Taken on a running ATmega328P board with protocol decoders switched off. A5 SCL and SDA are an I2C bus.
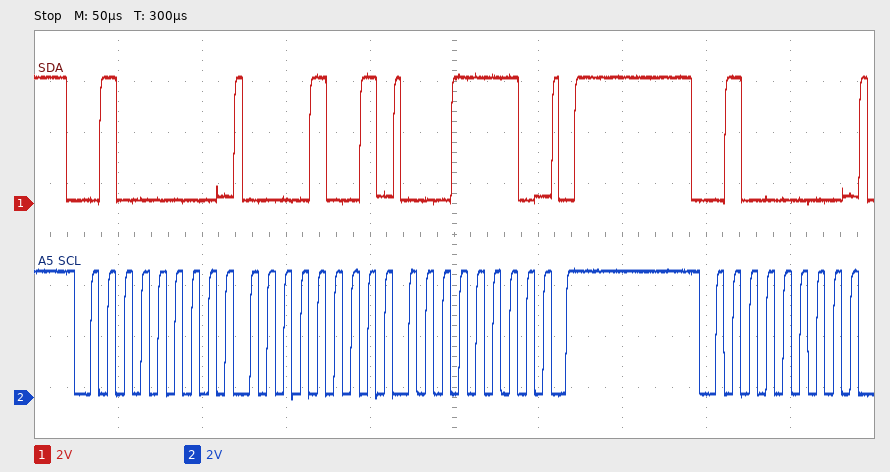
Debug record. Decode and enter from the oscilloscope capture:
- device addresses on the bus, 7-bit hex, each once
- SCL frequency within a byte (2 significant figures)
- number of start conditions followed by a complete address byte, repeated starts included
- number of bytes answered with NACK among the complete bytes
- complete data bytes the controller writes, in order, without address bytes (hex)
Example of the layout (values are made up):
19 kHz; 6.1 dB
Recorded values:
0x20; 100 kHz; 2; 0; 09 1E
